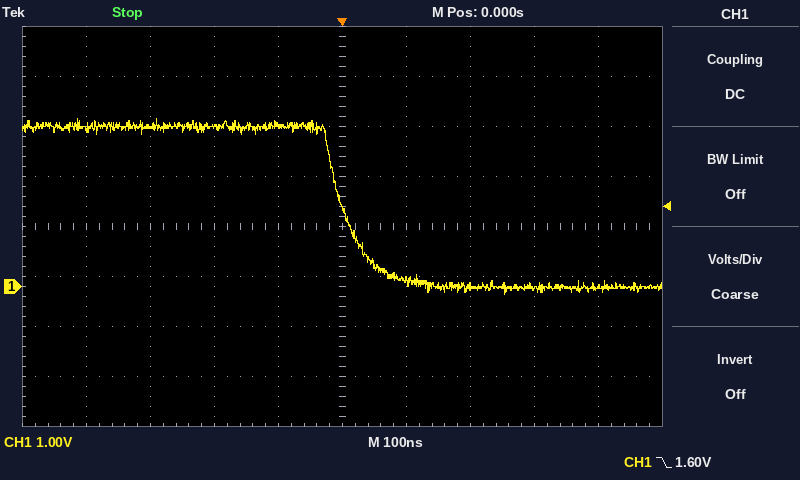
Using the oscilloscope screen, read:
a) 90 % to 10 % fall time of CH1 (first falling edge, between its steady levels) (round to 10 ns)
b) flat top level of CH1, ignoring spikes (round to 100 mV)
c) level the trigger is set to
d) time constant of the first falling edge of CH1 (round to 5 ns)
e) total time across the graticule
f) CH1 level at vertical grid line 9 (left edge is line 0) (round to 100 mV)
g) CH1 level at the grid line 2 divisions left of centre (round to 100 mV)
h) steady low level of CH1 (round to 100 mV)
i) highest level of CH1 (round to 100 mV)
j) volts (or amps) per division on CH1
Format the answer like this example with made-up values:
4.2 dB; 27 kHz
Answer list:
90 ns; 3.2 V; 1.60 V; 40 ns; 1 µs; 0.0 V; 3.2 V; 0.0 V; 3.4 V; 1 V
